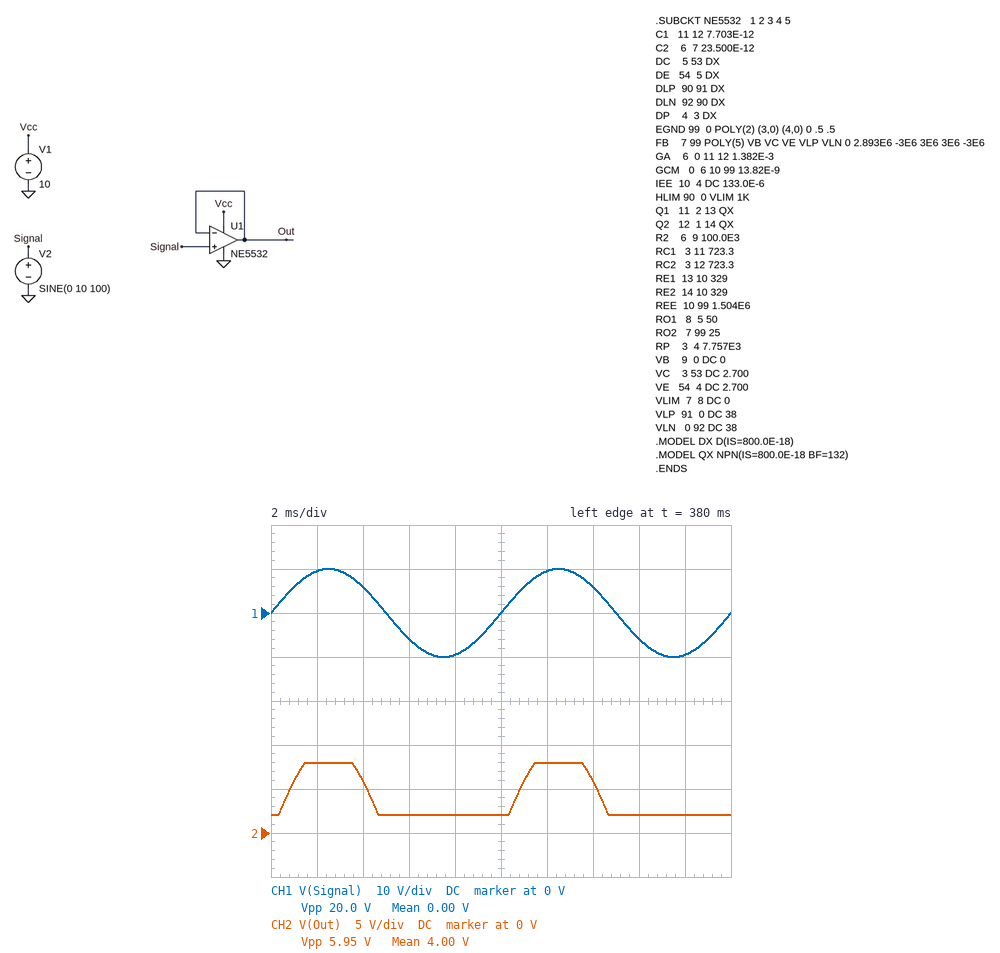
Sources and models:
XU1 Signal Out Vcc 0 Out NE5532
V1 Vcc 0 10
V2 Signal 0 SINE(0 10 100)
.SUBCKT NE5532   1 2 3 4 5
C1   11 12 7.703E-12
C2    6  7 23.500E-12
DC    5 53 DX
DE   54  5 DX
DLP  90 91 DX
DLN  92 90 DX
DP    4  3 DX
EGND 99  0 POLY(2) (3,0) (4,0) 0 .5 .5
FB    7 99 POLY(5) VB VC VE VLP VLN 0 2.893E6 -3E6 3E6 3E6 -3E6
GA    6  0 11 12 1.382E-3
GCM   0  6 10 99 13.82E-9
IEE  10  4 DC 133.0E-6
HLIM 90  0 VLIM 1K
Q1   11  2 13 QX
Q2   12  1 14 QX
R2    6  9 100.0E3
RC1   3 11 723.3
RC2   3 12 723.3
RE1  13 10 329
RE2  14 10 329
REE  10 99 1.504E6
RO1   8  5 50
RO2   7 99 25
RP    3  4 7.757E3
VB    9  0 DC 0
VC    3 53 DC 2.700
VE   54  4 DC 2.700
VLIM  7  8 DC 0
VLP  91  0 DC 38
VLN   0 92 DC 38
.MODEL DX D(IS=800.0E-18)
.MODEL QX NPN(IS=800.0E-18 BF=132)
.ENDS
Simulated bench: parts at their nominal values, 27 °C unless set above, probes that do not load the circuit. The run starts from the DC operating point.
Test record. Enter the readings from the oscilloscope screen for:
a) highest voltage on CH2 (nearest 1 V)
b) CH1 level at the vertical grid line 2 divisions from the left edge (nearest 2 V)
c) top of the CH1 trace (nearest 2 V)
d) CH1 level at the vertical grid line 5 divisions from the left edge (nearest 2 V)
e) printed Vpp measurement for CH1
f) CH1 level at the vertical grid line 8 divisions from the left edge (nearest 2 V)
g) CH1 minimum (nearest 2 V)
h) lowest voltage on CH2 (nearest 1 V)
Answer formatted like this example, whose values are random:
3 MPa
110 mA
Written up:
8 V
6 V
10 V
0 V
20.0 V
-6 V
-10 V
2 V
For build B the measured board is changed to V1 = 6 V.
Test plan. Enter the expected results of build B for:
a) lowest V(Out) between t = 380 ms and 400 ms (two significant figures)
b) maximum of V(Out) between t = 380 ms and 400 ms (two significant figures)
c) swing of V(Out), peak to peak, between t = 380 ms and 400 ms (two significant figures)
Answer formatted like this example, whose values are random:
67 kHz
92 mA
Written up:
1.9 V
4.0 V
2.0 V
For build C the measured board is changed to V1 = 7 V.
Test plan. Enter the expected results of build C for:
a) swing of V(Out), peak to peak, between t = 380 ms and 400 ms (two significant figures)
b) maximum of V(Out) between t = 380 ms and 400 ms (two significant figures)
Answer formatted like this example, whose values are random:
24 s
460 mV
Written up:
3.0 V
5.0 V
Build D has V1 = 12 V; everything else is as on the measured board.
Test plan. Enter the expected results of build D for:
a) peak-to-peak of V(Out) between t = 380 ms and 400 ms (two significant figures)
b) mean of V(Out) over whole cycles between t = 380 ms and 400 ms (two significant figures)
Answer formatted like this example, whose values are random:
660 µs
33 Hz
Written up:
7.9 V
4.3 V
